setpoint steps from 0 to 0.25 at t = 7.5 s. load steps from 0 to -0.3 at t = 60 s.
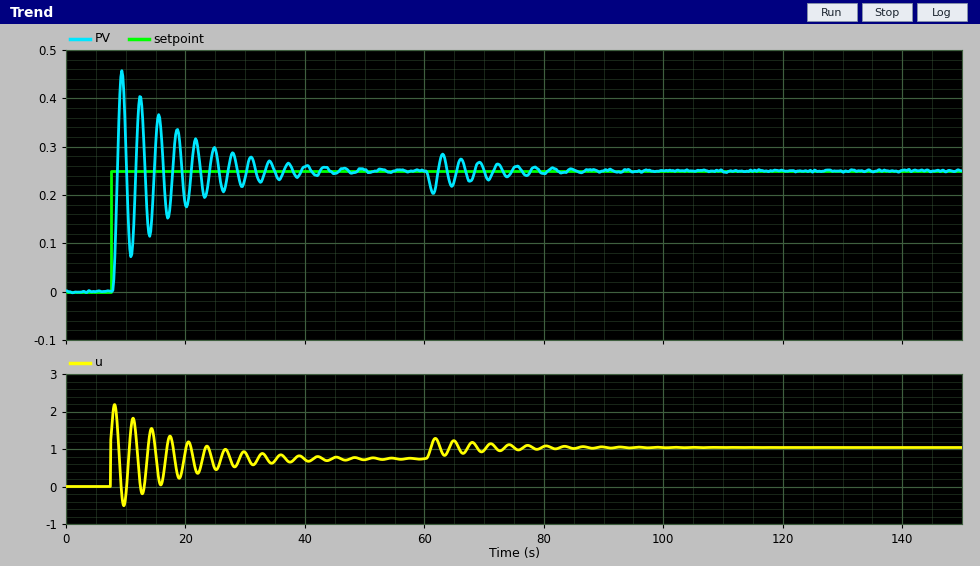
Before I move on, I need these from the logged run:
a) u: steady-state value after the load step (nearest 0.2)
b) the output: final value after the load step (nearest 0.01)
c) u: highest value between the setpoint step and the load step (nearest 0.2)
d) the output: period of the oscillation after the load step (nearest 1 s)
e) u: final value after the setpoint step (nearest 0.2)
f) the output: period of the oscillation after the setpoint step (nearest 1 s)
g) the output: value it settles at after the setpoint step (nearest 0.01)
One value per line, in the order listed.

1.0
0.25
2.2
3 s
0.8
3 s
0.25
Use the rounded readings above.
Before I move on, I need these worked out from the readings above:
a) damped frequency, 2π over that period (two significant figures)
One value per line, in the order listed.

2.1 rad/s
